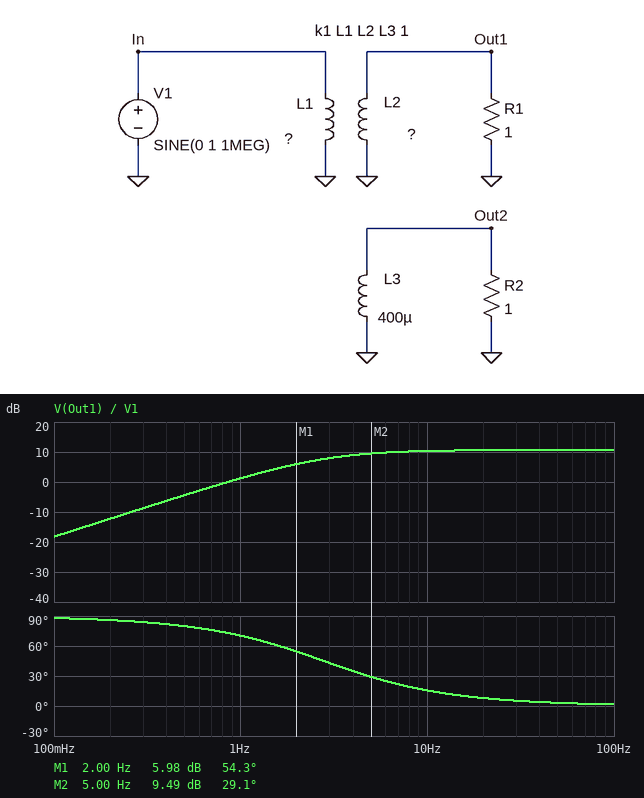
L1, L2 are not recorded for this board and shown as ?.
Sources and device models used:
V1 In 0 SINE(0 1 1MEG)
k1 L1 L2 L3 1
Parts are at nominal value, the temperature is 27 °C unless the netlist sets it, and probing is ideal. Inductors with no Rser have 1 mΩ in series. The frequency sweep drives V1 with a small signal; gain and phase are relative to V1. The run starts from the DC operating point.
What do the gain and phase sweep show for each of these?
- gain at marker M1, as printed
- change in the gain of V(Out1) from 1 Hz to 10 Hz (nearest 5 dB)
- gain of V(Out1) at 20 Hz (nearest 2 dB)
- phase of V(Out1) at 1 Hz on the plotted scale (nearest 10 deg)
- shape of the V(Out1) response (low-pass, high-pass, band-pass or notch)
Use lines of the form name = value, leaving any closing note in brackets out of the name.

gain at marker M1, as printed = 5.98 dB
change in the gain of V(Out1) from 1 Hz to 10 Hz = 10 dB
gain of V(Out1) at 20 Hz = 10 dB
phase of V(Out1) at 1 Hz on the plotted scale = 70 deg
shape of the V(Out1) response = high-pass
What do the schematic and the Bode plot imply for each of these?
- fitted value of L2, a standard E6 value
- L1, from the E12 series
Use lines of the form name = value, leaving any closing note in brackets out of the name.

fitted value of L2, a standard E6 value = 680 µH
L1, from the E12 series = 56 µH
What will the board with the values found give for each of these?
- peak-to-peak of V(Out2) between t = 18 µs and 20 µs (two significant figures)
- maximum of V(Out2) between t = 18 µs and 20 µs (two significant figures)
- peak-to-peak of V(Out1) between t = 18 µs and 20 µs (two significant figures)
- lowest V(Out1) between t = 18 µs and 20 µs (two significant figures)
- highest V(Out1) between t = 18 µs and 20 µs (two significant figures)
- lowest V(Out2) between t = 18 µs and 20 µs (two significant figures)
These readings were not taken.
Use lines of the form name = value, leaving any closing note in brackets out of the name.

peak-to-peak of V(Out2) between t = 18 µs and 20 µs = 5.2 V
maximum of V(Out2) between t = 18 µs and 20 µs = 2.6 V
peak-to-peak of V(Out1) between t = 18 µs and 20 µs = 6.8 V
lowest V(Out1) between t = 18 µs and 20 µs = -3.4 V
highest V(Out1) between t = 18 µs and 20 µs = 3.4 V
lowest V(Out2) between t = 18 µs and 20 µs = -2.6 V
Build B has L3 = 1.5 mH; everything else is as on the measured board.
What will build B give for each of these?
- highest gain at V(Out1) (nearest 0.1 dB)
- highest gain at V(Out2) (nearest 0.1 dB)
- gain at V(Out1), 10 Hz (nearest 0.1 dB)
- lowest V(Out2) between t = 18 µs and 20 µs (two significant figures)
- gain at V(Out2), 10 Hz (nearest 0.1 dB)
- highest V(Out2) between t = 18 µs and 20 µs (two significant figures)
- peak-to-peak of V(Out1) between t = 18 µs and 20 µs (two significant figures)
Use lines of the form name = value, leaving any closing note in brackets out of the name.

highest gain at V(Out1) = 10.5 dB
highest gain at V(Out2) = 13.9 dB
gain at V(Out1), 10 Hz = 10.2 dB
lowest V(Out2) between t = 18 µs and 20 µs = -5.0 V
gain at V(Out2), 10 Hz = 13.6 dB
highest V(Out2) between t = 18 µs and 20 µs = 5.0 V
peak-to-peak of V(Out1) between t = 18 µs and 20 µs = 6.7 V
